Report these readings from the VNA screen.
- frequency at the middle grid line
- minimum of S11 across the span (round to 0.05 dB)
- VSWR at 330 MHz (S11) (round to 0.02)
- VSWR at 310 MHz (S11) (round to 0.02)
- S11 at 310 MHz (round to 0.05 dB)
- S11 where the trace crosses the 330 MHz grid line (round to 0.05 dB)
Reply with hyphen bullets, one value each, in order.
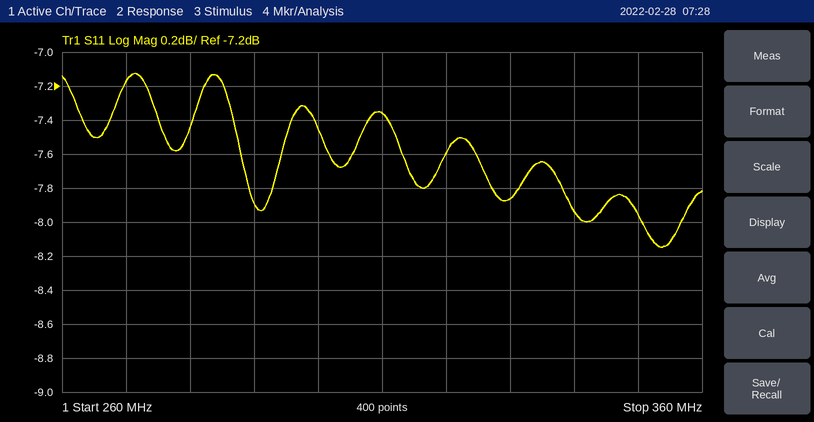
- 310 MHz
- -8.15 dB
- 2.36
- 2.50
- -7.35 dB
- -7.85 dB
